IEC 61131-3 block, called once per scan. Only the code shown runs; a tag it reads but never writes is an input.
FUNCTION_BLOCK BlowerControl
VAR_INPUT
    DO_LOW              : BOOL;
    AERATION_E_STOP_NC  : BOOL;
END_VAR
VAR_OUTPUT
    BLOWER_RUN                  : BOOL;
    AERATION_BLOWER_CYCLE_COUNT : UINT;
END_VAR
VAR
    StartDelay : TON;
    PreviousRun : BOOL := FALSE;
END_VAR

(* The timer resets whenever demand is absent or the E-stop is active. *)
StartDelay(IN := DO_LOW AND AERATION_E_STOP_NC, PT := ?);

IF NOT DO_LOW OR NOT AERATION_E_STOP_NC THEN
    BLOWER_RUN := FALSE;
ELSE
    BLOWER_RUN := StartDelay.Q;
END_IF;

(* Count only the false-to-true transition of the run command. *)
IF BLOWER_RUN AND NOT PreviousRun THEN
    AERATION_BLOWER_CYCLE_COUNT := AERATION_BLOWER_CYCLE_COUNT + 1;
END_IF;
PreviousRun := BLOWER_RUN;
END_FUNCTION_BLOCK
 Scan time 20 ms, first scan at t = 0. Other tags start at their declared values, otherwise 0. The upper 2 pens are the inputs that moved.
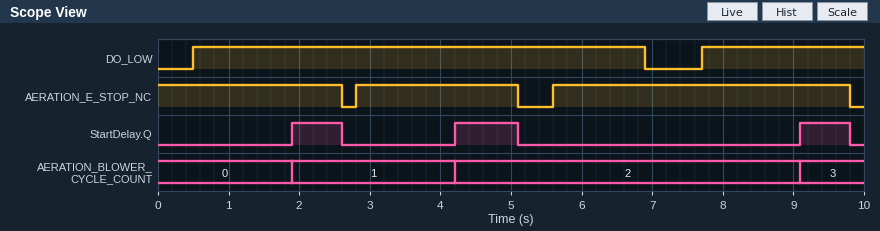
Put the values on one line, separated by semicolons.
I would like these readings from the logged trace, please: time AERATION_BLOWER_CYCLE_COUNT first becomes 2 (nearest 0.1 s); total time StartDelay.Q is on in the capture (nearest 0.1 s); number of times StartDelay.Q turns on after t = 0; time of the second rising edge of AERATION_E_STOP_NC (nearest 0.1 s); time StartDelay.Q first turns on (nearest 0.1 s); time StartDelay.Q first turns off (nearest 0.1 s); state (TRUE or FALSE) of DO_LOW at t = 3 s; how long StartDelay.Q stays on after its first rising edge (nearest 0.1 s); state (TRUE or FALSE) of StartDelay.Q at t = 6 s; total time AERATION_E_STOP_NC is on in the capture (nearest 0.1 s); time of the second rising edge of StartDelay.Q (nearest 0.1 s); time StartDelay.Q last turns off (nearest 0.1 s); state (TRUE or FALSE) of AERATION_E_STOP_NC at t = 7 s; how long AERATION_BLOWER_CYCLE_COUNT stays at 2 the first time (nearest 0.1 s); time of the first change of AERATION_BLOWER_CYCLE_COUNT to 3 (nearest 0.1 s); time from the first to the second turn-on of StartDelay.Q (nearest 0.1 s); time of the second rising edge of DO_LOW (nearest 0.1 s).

4.2 s; 2.3 s; 3; 5.6 s; 1.9 s; 2.6 s; TRUE; 0.7 s; FALSE; 9.1 s; 4.2 s; 9.8 s; TRUE; 4.9 s; 9.1 s; 2.3 s; 7.7 s
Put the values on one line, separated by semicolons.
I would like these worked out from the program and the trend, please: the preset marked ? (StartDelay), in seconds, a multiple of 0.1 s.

1.4 s
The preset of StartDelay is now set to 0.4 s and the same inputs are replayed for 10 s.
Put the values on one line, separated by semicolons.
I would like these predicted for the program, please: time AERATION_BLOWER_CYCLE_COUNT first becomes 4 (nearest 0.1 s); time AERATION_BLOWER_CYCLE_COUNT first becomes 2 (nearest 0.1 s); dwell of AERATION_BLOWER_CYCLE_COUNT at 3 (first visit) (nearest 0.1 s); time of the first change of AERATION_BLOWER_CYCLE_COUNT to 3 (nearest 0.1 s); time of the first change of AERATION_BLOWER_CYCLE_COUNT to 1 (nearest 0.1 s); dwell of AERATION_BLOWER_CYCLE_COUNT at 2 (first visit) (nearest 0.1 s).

8.1 s; 3.2 s; 2.1 s; 6.0 s; 0.9 s; 2.8 s
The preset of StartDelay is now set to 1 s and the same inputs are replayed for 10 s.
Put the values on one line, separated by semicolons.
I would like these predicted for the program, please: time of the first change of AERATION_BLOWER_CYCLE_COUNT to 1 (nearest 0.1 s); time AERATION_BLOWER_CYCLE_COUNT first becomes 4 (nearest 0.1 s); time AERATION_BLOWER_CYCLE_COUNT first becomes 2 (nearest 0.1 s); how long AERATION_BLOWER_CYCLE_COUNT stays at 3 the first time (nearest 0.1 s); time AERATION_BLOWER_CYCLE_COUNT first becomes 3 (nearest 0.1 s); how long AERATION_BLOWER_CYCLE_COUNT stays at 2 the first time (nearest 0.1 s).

1.5 s; 8.7 s; 3.8 s; 2.1 s; 6.6 s; 2.8 s
